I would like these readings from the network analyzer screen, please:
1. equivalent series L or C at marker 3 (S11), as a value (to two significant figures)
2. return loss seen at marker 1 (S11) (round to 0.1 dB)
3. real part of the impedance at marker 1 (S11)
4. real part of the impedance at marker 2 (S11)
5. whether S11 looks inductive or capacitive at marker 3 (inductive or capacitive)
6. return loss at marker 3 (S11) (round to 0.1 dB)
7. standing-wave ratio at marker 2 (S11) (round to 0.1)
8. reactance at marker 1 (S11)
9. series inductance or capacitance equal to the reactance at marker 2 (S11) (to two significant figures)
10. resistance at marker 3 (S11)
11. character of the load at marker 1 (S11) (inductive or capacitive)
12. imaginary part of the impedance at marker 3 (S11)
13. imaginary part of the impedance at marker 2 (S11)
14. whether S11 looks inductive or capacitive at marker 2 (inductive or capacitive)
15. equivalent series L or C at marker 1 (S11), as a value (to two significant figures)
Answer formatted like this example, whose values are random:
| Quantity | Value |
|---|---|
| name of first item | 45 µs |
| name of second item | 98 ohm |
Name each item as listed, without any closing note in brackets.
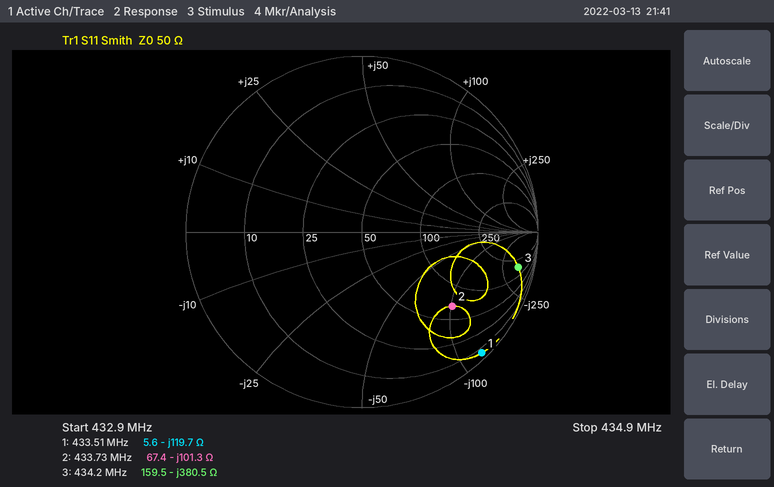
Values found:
| Quantity | Value |
|---|---|
| equivalent series L or C at marker 3 (S11), as a value | 960 fF |
| return loss seen at marker 1 (S11) | 0.3 dB |
| real part of the impedance at marker 1 | 5.6 Ω |
| real part of the impedance at marker 2 | 67.4 Ω |
| whether S11 looks inductive or capacitive at marker 3 | capacitive |
| return loss at marker 3 (S11) | 0.8 dB |
| standing-wave ratio at marker 2 (S11) | 4.9 |
| reactance at marker 1 | -119.7 Ω |
| series inductance or capacitance equal to the reactance at marker 2 (S11) | 3.6 pF |
| resistance at marker 3 | 159.5 Ω |
| character of the load at marker 1 (S11) | capacitive |
| imaginary part of the impedance at marker 3 | -380.5 Ω |
| imaginary part of the impedance at marker 2 | -101.3 Ω |
| whether S11 looks inductive or capacitive at marker 2 | capacitive |
| equivalent series L or C at marker 1 (S11), as a value | 3.1 pF |
